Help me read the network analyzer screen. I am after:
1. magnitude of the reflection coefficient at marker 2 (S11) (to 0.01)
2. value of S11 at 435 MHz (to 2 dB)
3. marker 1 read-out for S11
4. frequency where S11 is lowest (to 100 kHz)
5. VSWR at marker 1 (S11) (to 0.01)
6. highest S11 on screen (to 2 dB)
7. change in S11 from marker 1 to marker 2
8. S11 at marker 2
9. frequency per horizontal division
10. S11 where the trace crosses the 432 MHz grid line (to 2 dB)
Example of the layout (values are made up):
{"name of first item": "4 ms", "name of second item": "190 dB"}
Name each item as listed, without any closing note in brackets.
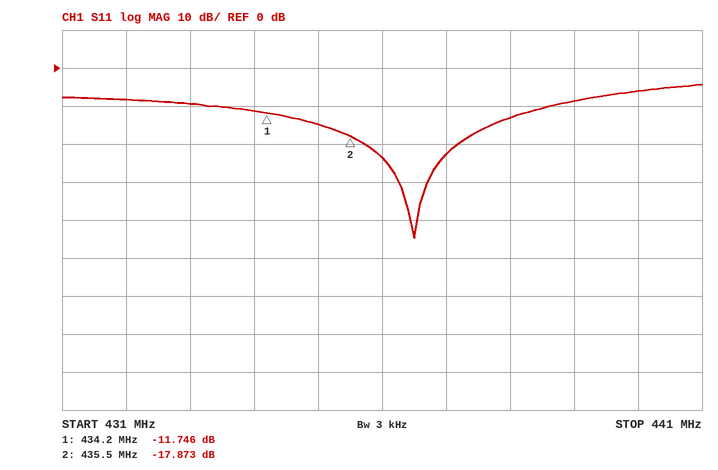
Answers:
{"magnitude of the reflection coefficient at marker 2 (S11)": "0.13", "value of S11 at 435 MHz": "-14 dB", "marker 1 read-out for S11": "-11.746 dB", "frequency where S11 is lowest": "436.5 MHz", "VSWR at marker 1 (S11)": "1.70", "highest S11 on screen": "-4 dB", "change in S11 from marker 1 to marker 2": "-6.127 dB", "S11 at marker 2": "-17.873 dB", "frequency per horizontal division": "1 MHz", "S11 where the trace crosses the 432 MHz grid line": "-8 dB"}
